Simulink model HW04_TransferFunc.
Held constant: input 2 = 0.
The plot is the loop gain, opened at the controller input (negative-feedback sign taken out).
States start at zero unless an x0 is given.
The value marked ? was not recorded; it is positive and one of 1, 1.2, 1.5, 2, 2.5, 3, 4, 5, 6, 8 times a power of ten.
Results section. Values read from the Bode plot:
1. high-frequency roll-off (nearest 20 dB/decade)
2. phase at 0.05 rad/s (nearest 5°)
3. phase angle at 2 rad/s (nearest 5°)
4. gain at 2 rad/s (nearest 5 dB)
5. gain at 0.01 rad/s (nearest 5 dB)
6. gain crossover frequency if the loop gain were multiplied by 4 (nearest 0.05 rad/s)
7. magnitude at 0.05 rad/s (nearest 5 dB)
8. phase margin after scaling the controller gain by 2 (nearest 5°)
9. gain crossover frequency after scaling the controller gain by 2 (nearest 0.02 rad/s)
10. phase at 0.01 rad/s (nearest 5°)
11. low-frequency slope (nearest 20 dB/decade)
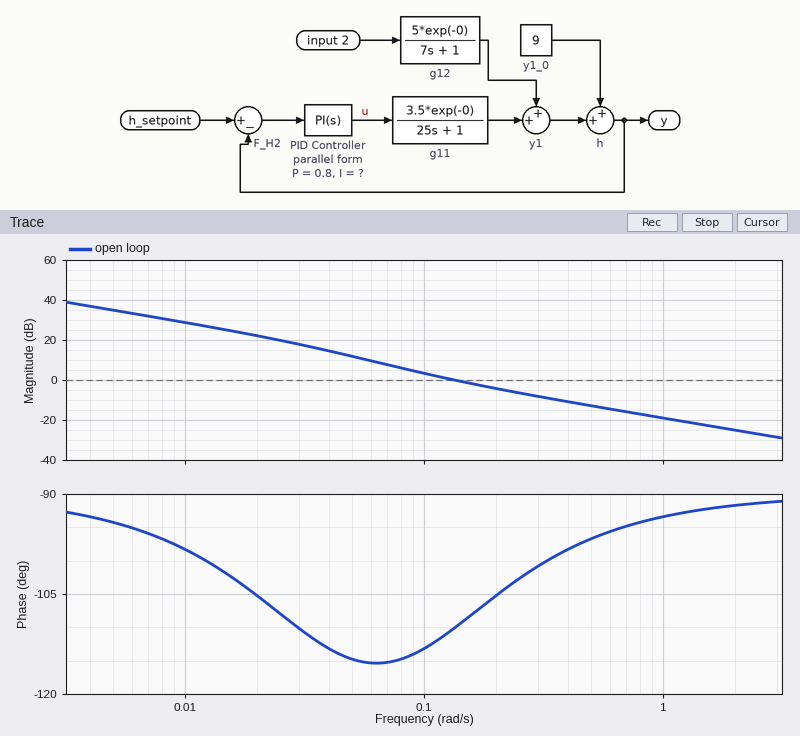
-20 dB/decade
-115°
-90°
-25 dB
30 dB
0.45 rad/s
10 dB
75°
0.24 rad/s
-100°
-20 dB/decade
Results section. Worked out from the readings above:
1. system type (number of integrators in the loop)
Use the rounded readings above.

1
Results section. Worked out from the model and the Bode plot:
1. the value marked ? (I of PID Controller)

0.08
